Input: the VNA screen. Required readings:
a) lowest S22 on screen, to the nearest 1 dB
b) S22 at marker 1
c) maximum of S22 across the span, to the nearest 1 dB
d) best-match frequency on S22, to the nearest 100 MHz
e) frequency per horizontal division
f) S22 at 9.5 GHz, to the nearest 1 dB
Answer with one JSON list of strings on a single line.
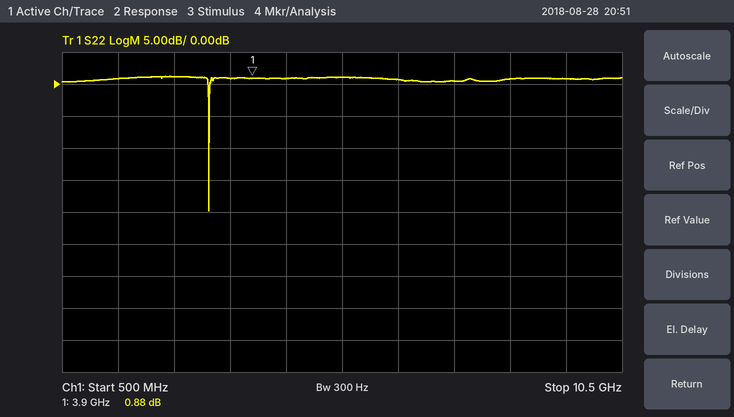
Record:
["-20 dB", "0.88 dB", "1 dB", "3.1 GHz", "1 GHz", "1 dB"]
